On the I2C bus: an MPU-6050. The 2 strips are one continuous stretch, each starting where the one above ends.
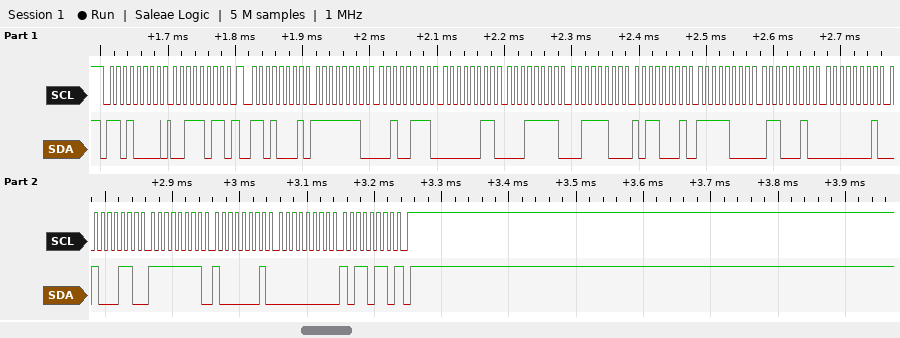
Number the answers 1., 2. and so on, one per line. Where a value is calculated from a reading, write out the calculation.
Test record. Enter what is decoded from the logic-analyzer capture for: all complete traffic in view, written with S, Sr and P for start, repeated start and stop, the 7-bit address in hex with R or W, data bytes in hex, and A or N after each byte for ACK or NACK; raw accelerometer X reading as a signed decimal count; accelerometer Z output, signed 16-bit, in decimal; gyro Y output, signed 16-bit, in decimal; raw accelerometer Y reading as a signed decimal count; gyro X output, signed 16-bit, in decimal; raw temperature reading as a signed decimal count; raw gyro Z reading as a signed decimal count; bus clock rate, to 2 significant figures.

1. S 68W A 3B A Sr 68R A FE A 27 A 03 A 1F A 3C A B1 A F8 A 62 A 01 A 46 A FF A 81 A 00 A B6 N P
2. 0xFE27 = -473
3. 0x3CB1 = 15537
4. 0xFF81 = -127
5. 0x031F = 799
6. 0x0146 = 326
7. 0xF862 = -1950
8. 0x00B6 = 182
9. 100 kHz
